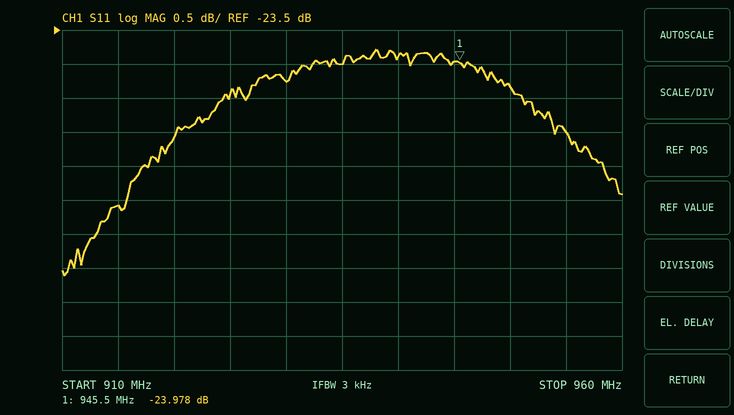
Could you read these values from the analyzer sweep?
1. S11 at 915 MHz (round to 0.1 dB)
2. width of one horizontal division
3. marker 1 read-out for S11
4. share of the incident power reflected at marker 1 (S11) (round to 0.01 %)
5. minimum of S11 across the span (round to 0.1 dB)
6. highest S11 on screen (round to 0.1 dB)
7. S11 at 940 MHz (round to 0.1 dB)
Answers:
-26.1 dB
5 MHz
-23.978 dB
0.40 %
-27.1 dB
-23.8 dB
-23.9 dB
